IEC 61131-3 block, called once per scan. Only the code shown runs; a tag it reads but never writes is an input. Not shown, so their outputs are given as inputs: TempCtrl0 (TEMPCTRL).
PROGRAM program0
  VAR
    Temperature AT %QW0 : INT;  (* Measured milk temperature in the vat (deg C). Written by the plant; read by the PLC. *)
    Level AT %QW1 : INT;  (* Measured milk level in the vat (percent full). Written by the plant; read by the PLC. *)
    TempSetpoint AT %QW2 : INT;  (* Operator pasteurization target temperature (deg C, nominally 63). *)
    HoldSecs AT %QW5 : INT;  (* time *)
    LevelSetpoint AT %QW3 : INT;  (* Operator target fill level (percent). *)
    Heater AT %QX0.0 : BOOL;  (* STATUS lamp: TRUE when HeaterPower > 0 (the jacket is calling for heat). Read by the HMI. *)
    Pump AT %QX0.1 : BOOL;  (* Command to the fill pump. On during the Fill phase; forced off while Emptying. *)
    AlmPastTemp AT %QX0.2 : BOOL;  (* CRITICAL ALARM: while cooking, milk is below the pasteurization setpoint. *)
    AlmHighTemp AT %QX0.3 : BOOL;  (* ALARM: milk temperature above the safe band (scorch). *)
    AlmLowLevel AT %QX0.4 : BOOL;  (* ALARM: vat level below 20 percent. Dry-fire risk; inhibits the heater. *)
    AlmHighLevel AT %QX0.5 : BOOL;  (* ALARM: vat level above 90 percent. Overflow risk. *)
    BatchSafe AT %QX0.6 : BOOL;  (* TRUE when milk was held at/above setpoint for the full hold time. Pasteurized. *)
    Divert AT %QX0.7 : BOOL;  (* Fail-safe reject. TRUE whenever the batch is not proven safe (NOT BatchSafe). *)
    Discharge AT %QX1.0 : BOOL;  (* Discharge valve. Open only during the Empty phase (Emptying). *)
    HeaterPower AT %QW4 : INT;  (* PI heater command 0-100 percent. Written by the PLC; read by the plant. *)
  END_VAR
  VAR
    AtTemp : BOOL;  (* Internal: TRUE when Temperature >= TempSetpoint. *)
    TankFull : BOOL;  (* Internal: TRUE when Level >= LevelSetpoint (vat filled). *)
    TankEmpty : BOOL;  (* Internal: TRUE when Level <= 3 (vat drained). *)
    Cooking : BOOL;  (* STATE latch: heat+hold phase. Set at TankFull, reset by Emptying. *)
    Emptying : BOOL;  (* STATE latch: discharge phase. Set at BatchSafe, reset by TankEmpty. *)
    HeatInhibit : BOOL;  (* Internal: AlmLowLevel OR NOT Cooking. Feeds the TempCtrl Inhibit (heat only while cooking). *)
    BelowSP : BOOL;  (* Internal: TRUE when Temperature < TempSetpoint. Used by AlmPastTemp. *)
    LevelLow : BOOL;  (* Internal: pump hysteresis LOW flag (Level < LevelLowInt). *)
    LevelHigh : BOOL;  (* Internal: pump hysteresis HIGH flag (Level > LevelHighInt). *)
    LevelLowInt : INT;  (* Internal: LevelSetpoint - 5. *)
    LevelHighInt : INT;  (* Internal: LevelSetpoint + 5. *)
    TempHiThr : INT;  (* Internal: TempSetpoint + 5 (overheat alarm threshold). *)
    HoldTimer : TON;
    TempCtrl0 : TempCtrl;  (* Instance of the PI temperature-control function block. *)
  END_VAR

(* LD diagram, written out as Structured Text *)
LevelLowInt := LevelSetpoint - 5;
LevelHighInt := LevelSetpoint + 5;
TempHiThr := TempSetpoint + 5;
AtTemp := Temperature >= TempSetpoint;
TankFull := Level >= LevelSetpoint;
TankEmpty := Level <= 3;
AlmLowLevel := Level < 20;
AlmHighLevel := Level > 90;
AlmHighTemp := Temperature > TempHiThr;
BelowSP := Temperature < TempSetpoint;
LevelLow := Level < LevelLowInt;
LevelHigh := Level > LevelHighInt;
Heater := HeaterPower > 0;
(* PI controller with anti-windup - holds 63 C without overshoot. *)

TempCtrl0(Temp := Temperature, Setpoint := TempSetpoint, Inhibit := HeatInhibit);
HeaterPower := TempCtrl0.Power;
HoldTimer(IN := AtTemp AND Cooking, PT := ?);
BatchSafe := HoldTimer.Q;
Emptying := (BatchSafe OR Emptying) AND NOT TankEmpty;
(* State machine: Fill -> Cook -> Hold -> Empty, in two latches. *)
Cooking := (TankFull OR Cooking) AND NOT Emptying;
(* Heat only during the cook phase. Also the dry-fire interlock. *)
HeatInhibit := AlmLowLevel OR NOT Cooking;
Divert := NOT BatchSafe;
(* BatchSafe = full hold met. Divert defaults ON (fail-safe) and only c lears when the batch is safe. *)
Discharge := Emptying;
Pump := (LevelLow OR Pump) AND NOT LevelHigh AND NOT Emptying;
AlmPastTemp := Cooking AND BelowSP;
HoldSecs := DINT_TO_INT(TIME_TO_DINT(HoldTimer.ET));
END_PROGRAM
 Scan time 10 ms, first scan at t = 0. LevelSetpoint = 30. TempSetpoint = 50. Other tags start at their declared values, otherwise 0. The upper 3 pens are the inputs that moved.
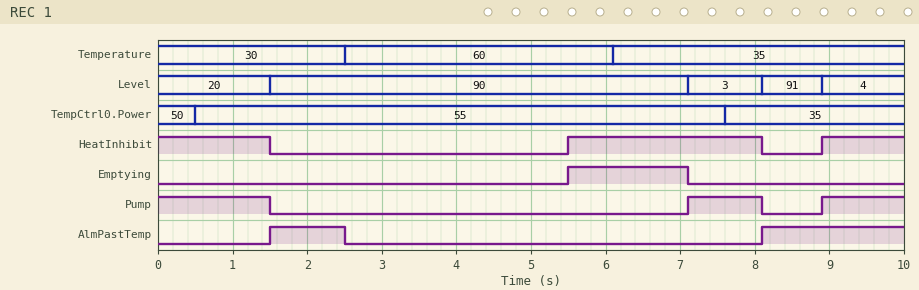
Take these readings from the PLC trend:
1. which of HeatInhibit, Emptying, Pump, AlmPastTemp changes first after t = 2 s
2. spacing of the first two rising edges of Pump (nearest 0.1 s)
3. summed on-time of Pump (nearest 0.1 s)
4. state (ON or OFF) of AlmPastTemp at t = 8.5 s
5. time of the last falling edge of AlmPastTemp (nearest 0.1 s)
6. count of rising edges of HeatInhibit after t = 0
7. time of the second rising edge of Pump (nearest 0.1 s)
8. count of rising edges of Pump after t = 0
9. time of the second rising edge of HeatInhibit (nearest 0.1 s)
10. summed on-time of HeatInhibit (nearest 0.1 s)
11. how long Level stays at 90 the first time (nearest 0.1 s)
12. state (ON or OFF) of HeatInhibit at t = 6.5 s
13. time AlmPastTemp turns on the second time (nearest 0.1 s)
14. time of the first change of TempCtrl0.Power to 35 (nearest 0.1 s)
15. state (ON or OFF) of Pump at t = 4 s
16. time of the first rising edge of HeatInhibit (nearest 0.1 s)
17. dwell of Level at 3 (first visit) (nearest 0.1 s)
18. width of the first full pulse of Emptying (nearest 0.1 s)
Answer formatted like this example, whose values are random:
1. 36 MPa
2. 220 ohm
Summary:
1. AlmPastTemp
2. 1.8 s
3. 3.6 s
4. ON
5. 2.5 s
6. 2
7. 8.9 s
8. 2
9. 8.9 s
10. 5.2 s
11. 5.6 s
12. ON
13. 8.1 s
14. 7.6 s
15. OFF
16. 5.5 s
17. 1.0 s
18. 1.6 s
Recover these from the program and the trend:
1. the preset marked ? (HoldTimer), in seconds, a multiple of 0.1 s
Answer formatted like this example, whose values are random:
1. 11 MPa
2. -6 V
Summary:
1. 3.0 s
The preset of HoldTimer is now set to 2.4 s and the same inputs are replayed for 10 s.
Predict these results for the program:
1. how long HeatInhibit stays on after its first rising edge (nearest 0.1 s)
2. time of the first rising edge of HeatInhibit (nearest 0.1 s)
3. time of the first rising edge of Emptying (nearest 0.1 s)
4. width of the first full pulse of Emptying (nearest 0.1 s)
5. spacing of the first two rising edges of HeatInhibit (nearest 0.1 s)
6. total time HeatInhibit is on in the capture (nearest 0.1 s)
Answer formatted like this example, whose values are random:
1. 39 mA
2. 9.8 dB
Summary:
1. 3.2 s
2. 4.9 s
3. 4.9 s
4. 2.2 s
5. 4.0 s
6. 5.8 s
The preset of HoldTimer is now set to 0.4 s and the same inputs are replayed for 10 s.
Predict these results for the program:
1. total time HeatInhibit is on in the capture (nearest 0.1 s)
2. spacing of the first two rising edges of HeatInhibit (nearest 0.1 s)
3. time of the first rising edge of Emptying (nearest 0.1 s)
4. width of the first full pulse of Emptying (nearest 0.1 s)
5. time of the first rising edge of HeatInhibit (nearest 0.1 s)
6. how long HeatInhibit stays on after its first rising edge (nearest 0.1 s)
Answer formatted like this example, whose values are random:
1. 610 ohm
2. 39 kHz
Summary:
1. 7.8 s
2. 6.0 s
3. 2.9 s
4. 4.2 s
5. 2.9 s
6. 5.2 s
